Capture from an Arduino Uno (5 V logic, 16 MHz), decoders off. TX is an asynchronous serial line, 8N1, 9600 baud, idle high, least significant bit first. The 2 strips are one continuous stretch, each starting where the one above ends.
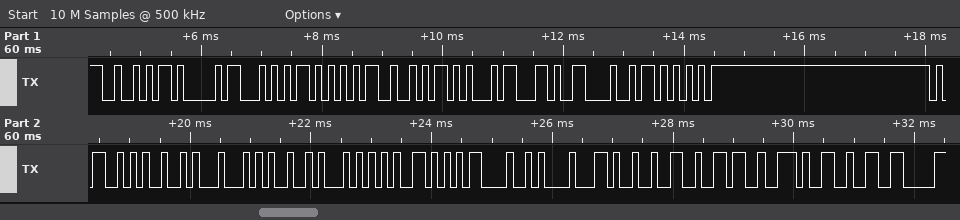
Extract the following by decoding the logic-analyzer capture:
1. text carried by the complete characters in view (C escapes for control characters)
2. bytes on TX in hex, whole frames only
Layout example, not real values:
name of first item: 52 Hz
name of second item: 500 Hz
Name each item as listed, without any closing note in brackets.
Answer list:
text carried by the complete characters in view: "RATURE,HUMIDITY\r\n,26.2"
bytes on TX in hex, whole frames only: 0x52 0x41 0x54 0x55 0x52 0x45 0x2C 0x48 0x55 0x4D 0x49 0x44 0x49 0x54 0x59 0x0D 0x0A 0x2C 0x32 0x36 0x2E 0x32
